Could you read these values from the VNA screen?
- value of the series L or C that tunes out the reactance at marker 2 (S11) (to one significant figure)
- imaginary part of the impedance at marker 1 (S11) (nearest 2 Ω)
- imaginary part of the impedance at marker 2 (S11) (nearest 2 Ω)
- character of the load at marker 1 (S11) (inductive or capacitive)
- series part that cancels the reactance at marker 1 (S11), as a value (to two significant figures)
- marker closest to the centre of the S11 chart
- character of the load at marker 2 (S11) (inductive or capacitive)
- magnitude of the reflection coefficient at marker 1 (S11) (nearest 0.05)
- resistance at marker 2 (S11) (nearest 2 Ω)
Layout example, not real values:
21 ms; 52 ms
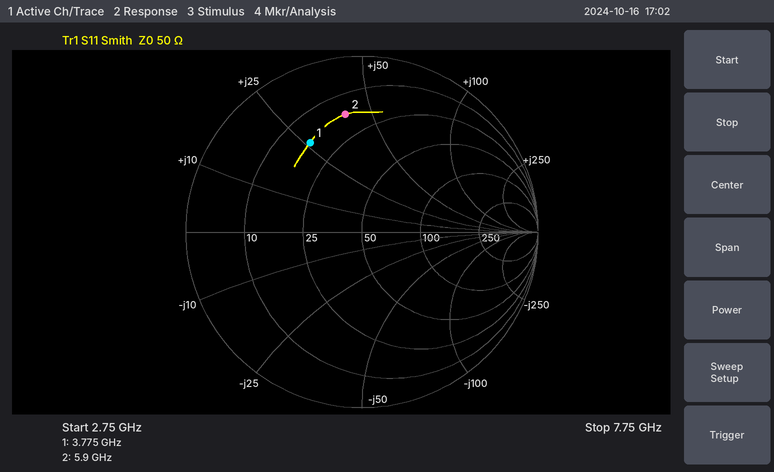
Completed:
700 fF; +26 Ω; +40 Ω; inductive; 1.6 pF; marker 1; inductive; 0.60; 16 Ω
